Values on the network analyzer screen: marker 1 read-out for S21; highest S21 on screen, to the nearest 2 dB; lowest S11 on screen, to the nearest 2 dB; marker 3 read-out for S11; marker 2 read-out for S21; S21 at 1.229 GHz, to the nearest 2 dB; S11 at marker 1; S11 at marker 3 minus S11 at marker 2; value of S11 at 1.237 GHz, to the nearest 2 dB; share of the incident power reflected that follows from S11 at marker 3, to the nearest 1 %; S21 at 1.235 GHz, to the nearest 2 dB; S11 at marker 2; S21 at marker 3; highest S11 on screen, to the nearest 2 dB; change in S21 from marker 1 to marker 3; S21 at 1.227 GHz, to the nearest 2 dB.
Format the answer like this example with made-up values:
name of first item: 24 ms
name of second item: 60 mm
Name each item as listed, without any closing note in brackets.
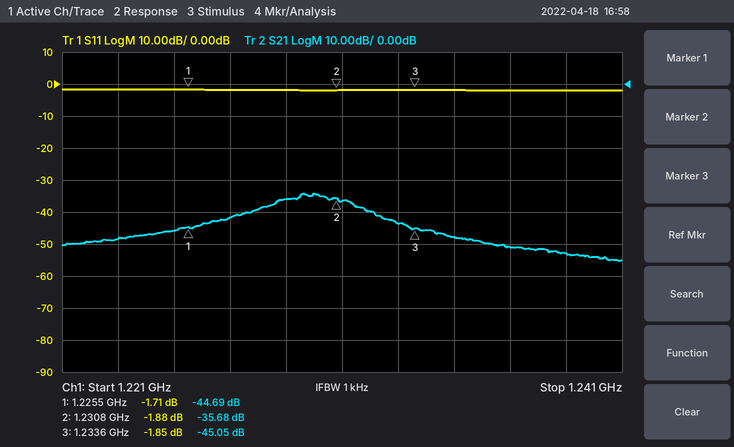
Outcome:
marker 1 read-out for S21: -44.69 dB
highest S21 on screen, to the nearest 2 dB: -34 dB
lowest S11 on screen, to the nearest 2 dB: -2 dB
marker 3 read-out for S11: -1.85 dB
marker 2 read-out for S21: -35.68 dB
S21 at 1.229 GHz, to the nearest 2 dB: -36 dB
S11 at marker 1: -1.71 dB
S11 at marker 3 minus S11 at marker 2: 0.03 dB
value of S11 at 1.237 GHz, to the nearest 2 dB: -2 dB
share of the incident power reflected that follows from S11 at marker 3, to the nearest 1 %: 65 %
S21 at 1.235 GHz, to the nearest 2 dB: -48 dB
S11 at marker 2: -1.88 dB
S21 at marker 3: -45.05 dB
highest S11 on screen, to the nearest 2 dB: -2 dB
change in S21 from marker 1 to marker 3: -0.36 dB
S21 at 1.227 GHz, to the nearest 2 dB: -42 dB
